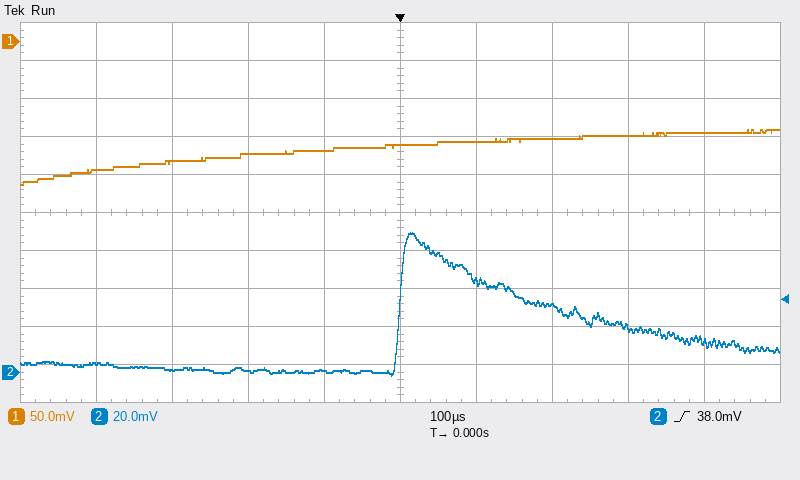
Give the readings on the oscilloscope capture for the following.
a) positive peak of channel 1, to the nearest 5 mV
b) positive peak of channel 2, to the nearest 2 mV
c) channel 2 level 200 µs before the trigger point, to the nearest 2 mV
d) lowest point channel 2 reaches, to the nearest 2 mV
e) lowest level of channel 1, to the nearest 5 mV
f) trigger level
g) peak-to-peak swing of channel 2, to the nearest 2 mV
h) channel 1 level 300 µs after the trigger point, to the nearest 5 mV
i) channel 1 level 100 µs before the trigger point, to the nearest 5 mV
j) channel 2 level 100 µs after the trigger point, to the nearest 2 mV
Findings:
-115 mV
74 mV
0 mV
-2 mV
-190 mV
38.0 mV
76 mV
-125 mV
-145 mV
48 mV
